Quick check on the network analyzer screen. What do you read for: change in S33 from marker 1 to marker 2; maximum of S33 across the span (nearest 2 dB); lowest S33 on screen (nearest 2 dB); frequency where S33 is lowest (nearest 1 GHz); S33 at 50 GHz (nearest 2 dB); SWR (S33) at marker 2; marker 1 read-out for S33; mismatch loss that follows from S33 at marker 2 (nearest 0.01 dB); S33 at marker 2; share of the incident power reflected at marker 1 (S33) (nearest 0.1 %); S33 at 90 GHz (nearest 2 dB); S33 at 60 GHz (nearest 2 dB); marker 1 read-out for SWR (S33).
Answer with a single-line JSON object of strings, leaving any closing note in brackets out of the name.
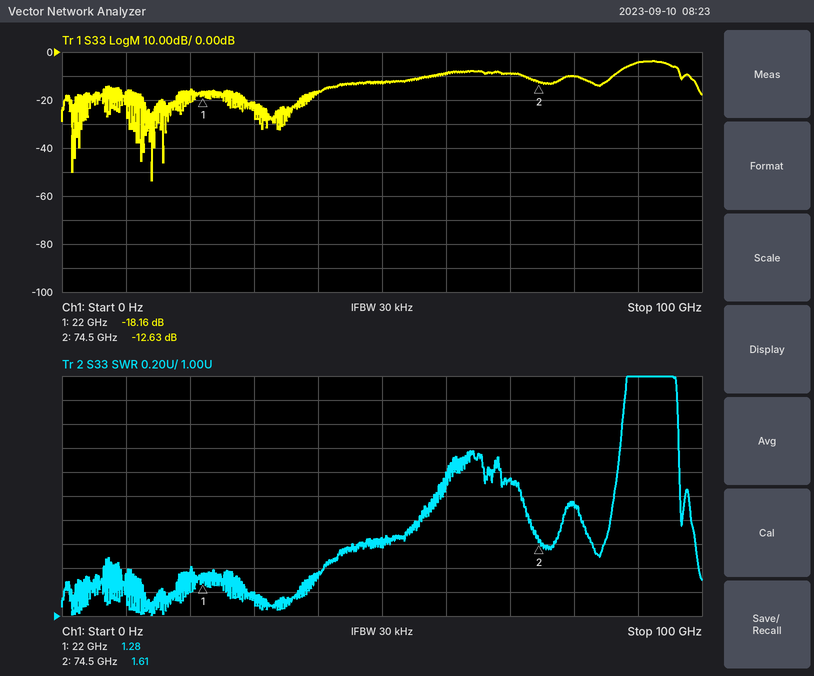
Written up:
{"change in S33 from marker 1 to marker 2": "5.53 dB", "maximum of S33 across the span": "-4 dB", "lowest S33 on screen": "-54 dB", "frequency where S33 is lowest": "14 GHz", "S33 at 50 GHz": "-12 dB", "SWR (S33) at marker 2": "1.61", "marker 1 read-out for S33": "-18.16 dB", "mismatch loss that follows from S33 at marker 2": "0.24 dB", "S33 at marker 2": "-12.63 dB", "share of the incident power reflected at marker 1 (S33)": "1.5 %", "S33 at 90 GHz": "-4 dB", "S33 at 60 GHz": "-8 dB", "marker 1 read-out for SWR": "1.28"}
